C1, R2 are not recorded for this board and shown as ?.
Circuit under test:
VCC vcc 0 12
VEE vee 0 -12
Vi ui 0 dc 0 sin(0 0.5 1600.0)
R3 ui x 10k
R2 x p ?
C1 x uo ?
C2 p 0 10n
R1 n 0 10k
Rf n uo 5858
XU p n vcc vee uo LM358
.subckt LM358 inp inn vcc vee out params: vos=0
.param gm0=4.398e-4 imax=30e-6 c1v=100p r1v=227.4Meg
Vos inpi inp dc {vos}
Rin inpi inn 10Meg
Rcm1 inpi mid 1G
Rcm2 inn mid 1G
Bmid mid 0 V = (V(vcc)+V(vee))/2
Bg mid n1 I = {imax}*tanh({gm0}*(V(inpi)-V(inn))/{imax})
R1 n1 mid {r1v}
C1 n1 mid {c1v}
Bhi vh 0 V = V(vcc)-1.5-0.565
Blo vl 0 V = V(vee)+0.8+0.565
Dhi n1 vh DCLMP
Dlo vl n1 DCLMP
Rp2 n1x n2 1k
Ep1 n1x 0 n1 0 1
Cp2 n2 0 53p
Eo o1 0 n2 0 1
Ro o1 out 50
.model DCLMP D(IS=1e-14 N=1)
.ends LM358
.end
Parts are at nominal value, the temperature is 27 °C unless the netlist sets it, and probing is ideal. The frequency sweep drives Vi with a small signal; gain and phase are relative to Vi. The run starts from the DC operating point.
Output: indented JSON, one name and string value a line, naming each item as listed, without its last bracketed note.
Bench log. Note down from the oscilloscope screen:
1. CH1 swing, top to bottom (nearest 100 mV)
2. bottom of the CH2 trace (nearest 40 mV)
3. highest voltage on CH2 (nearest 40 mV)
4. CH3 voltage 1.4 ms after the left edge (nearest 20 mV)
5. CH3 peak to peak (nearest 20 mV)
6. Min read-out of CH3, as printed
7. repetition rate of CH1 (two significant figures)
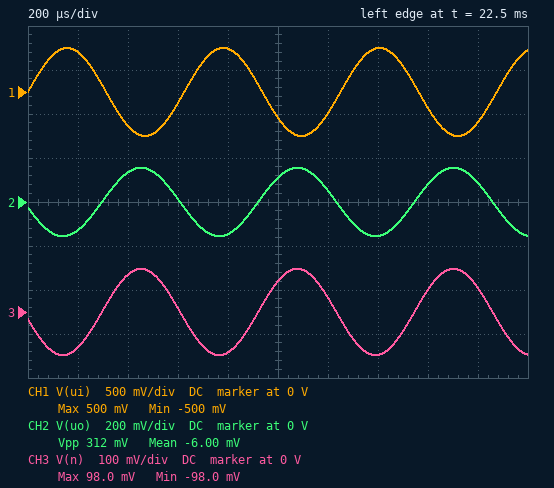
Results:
{
  "CH1 swing, top to bottom": "1.0 V",
  "bottom of the CH2 trace": "-160 mV",
  "highest voltage on CH2": "160 mV",
  "CH3 voltage 1.4 ms after the left edge": "-100 mV",
  "CH3 peak to peak": "200 mV",
  "Min read-out of CH3, as printed": "-98.0 mV",
  "repetition rate of CH1": "1.6 kHz"
}
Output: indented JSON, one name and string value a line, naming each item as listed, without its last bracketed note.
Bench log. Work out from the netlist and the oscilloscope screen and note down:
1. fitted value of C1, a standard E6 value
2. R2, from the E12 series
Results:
{
  "fitted value of C1, a standard E6 value": "33 nF",
  "R2, from the E12 series": "18 kΩ"
}
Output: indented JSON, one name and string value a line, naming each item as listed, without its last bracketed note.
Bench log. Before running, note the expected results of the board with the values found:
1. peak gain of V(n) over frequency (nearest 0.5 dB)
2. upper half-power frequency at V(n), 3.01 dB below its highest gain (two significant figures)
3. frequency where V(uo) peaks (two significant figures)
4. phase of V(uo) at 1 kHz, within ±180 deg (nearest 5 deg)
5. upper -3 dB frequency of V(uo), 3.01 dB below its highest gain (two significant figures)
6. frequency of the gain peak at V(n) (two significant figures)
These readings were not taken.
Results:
{
  "peak gain of V(n) over frequency": "9.0 dB",
  "upper half-power frequency at V(n), 3.01 dB below its highest gain": "740 Hz",
  "frequency where V(uo) peaks": "630 Hz",
  "phase of V(uo) at 1 kHz, within ±180 deg": "-160 deg",
  "upper -3 dB frequency of V(uo), 3.01 dB below its highest gain": "740 Hz",
  "frequency of the gain peak at V(n)": "630 Hz"
}
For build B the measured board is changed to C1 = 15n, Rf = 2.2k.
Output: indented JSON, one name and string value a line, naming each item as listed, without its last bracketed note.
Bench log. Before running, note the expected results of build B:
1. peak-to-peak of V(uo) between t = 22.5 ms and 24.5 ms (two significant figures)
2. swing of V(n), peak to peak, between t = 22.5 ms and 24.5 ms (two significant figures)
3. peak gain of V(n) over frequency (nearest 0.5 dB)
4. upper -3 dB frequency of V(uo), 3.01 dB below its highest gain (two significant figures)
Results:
{
  "peak-to-peak of V(uo) between t = 22.5 ms and 24.5 ms": "400 mV",
  "swing of V(n), peak to peak, between t = 22.5 ms and 24.5 ms": "330 mV",
  "peak gain of V(n) over frequency": "0 dB",
  "upper -3 dB frequency of V(uo), 3.01 dB below its highest gain": "910 Hz"
}
